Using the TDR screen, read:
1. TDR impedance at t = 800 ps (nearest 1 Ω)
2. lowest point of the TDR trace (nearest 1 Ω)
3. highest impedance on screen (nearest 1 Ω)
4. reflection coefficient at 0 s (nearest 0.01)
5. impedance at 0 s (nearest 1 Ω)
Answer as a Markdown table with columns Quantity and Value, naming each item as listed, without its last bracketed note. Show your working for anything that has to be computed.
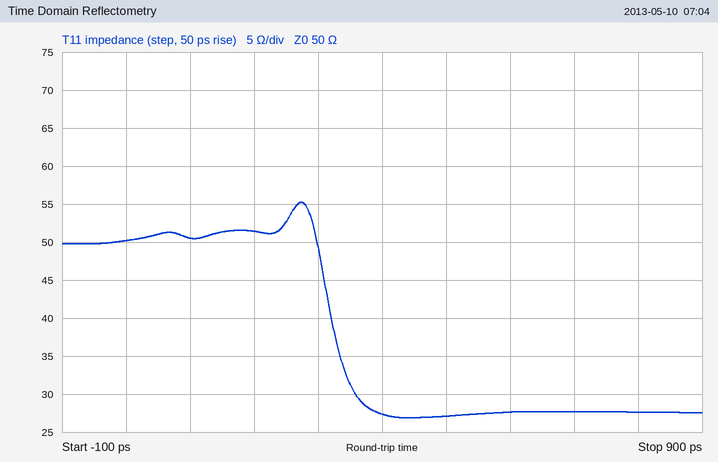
| Quantity | Value |
|---|---|
| TDR impedance at t = 800 ps | 28 Ω |
| lowest point of the TDR trace | 27 Ω |
| highest impedance on screen | 55 Ω |
| reflection coefficient at 0 s | (50 − 50)/(50 + 50) ≈ 0.00 |
| impedance at 0 s | 50 Ω |
